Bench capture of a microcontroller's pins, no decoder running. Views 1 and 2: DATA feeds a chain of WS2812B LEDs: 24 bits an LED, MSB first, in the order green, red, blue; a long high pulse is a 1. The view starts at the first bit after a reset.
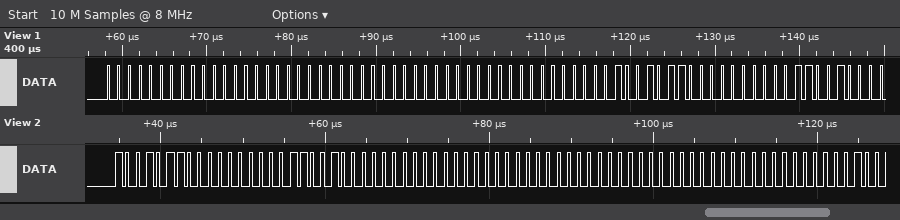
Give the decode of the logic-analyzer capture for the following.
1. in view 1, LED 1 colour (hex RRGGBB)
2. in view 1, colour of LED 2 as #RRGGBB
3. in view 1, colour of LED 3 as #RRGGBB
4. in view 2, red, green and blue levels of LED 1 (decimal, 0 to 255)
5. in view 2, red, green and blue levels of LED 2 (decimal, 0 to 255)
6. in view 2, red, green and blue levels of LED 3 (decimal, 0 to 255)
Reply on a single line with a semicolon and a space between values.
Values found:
#000000; #000000; #009664; 0, 150, 100; 0, 0, 0; 0, 0, 0
